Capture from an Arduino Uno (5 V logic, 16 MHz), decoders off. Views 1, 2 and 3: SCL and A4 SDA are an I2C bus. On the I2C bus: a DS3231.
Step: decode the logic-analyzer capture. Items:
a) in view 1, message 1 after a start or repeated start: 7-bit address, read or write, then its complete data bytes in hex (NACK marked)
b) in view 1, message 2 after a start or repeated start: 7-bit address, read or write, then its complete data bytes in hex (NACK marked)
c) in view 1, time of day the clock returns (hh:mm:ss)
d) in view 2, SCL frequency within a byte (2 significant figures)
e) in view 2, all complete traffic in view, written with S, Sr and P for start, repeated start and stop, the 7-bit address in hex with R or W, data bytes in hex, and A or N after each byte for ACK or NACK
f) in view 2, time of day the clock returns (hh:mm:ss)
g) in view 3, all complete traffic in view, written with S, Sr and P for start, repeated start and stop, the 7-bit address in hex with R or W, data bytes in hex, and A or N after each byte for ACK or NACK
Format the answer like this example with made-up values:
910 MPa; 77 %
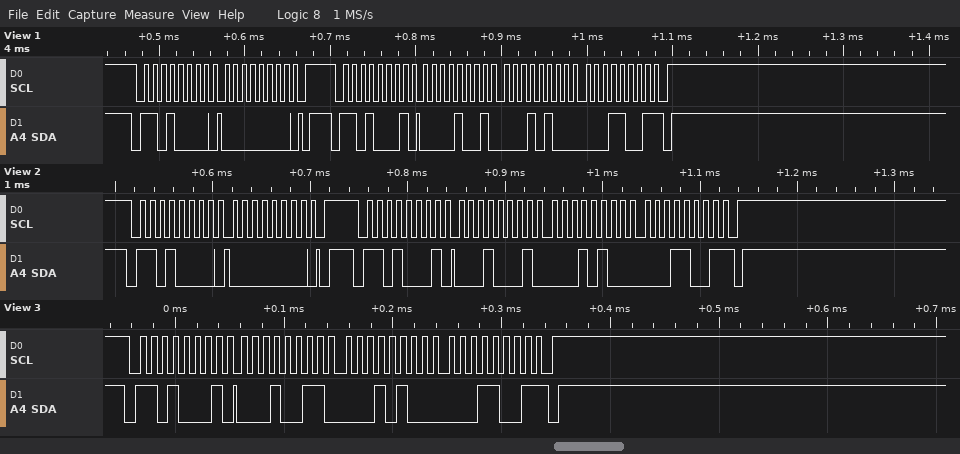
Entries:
0x68 write: 00; 0x68 read: 09 14 19 NACK; 19:14:09; 100 kHz; S 68W A 00 A P S 68R A 11 A 14 A 19 N P; 19:14:11; S 68R A 13 A 14 A 19 N P
